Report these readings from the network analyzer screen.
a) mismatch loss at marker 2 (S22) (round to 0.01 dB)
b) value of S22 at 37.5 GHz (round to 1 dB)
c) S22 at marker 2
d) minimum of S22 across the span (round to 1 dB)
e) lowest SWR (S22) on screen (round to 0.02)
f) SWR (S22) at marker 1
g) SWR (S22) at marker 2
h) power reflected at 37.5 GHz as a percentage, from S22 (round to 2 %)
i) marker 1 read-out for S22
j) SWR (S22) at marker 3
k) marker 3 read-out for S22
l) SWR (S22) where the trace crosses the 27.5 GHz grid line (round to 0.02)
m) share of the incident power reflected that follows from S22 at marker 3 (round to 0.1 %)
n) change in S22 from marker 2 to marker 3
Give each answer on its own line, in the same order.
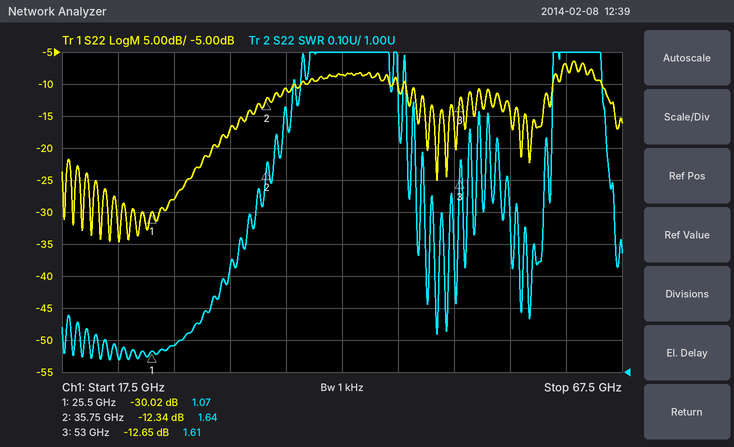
0.26 dB
-11 dB
-12.34 dB
-35 dB
1.04
1.07
1.64
8 %
-30.02 dB
1.61
-12.65 dB
1.08
5.4 %
-0.31 dB
